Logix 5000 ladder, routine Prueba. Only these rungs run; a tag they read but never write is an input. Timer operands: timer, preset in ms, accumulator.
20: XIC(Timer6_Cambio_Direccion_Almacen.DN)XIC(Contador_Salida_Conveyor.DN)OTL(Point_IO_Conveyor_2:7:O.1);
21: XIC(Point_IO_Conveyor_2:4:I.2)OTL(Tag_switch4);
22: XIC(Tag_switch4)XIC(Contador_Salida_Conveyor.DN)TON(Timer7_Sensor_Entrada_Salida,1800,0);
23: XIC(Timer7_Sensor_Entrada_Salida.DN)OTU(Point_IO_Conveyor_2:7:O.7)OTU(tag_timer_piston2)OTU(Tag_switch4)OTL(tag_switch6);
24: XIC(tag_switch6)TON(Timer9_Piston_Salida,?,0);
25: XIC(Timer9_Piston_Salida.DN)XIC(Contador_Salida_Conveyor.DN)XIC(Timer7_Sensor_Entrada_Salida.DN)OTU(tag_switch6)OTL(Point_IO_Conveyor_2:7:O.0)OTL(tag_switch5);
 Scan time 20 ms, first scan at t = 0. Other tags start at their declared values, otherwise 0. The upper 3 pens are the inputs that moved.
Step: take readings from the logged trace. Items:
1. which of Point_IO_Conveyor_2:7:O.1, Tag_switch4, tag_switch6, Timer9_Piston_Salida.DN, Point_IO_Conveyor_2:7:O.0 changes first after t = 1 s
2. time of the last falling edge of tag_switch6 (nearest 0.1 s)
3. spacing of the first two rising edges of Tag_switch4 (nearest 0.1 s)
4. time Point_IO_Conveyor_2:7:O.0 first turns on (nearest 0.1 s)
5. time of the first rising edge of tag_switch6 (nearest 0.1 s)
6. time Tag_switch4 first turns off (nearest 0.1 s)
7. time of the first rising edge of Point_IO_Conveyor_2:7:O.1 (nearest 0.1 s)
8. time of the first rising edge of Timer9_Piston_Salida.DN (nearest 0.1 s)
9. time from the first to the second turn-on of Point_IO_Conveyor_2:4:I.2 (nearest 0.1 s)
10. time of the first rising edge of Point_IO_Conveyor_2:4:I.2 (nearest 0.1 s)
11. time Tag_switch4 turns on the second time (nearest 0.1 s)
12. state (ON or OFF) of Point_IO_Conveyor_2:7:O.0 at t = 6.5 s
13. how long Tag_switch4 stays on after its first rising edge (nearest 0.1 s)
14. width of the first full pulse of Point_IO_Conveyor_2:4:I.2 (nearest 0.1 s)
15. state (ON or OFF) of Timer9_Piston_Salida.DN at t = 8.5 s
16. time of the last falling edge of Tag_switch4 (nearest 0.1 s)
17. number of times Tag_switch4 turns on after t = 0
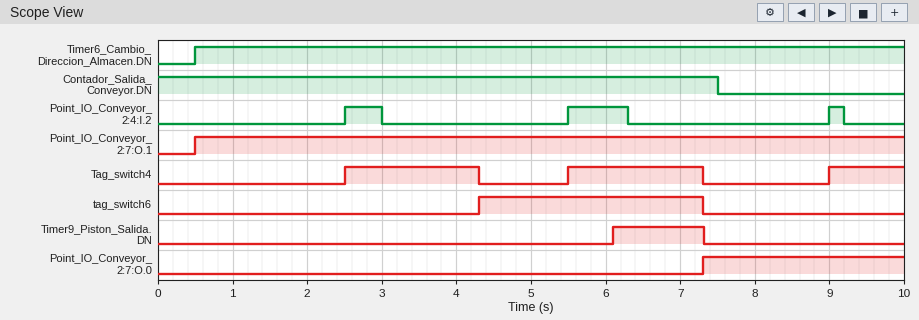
Tag_switch4
7.3 s
3.0 s
7.3 s
4.3 s
4.3 s
0.5 s
6.1 s
3.0 s
2.5 s
5.5 s
OFF
1.8 s
0.5 s
OFF
7.3 s
3
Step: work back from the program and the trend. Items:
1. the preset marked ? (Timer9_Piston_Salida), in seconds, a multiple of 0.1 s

1.8 s
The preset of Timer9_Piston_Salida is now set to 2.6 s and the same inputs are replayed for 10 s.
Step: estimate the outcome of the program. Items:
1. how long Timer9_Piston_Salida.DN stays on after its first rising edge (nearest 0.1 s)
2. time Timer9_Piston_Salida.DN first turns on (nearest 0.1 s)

0.4 s
6.9 s
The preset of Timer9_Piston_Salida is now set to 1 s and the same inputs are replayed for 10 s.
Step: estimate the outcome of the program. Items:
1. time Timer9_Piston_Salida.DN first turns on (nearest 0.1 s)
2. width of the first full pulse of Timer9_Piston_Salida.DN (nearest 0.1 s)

5.3 s
2.0 s
